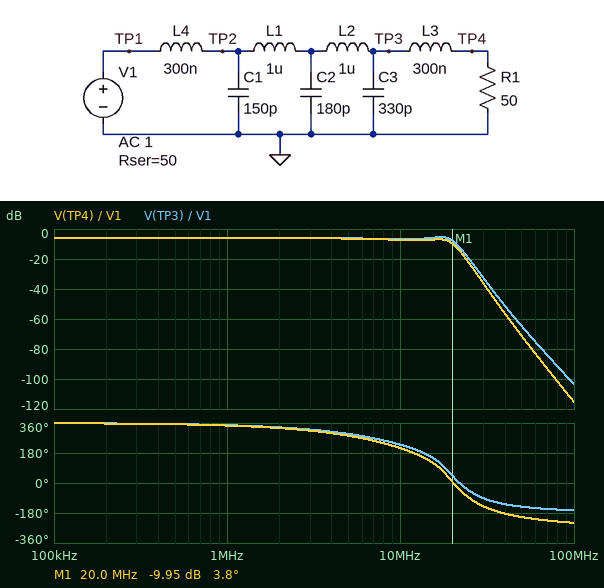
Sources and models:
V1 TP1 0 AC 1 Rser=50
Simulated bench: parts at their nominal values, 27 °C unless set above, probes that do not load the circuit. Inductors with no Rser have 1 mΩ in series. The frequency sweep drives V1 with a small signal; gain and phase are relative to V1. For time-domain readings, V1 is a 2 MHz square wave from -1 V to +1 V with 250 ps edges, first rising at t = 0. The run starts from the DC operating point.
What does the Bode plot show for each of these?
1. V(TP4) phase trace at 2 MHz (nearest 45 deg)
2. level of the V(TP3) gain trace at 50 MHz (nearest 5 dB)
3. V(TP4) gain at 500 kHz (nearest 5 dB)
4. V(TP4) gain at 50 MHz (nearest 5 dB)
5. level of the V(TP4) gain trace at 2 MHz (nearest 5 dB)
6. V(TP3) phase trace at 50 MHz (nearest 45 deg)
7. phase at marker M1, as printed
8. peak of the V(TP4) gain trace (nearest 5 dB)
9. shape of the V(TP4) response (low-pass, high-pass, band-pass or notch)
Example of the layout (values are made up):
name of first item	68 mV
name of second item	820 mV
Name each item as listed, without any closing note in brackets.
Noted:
V(TP4) phase trace at 2 MHz	315 deg
level of the V(TP3) gain trace at 50 MHz	-65 dB
V(TP4) gain at 500 kHz	-5 dB
V(TP4) gain at 50 MHz	-70 dB
level of the V(TP4) gain trace at 2 MHz	-5 dB
V(TP3) phase trace at 50 MHz	-135 deg
phase at marker M1, as printed	3.8 deg
peak of the V(TP4) gain trace	-5 dB
shape of the V(TP4) response	low-pass
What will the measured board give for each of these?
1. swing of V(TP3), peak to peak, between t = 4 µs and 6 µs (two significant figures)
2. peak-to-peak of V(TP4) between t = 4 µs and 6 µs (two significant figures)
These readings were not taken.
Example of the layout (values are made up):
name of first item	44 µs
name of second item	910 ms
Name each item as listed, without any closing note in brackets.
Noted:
swing of V(TP3), peak to peak, between t = 4 µs and 6 µs	1.3 V
peak-to-peak of V(TP4) between t = 4 µs and 6 µs	1.2 V
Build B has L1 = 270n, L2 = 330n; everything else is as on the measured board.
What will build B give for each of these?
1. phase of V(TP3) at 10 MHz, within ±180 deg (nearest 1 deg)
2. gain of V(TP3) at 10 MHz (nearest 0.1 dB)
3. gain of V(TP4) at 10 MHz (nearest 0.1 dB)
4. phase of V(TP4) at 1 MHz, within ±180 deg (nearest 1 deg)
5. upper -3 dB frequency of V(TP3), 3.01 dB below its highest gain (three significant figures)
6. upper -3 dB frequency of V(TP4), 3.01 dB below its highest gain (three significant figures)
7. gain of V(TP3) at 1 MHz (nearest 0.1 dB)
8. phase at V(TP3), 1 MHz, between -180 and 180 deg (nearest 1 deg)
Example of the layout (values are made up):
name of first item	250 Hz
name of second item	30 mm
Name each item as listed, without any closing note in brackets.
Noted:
phase of V(TP3) at 10 MHz, within ±180 deg	-83 deg
gain of V(TP3) at 10 MHz	-6.1 dB
gain of V(TP4) at 10 MHz	-6.7 dB
phase of V(TP4) at 1 MHz, within ±180 deg	-10 deg
upper -3 dB frequency of V(TP3), 3.01 dB below its highest gain	26.8 MHz
upper -3 dB frequency of V(TP4), 3.01 dB below its highest gain	25.7 MHz
gain of V(TP3) at 1 MHz	-6.0 dB
phase at V(TP3), 1 MHz, between -180 and 180 deg	-8 deg
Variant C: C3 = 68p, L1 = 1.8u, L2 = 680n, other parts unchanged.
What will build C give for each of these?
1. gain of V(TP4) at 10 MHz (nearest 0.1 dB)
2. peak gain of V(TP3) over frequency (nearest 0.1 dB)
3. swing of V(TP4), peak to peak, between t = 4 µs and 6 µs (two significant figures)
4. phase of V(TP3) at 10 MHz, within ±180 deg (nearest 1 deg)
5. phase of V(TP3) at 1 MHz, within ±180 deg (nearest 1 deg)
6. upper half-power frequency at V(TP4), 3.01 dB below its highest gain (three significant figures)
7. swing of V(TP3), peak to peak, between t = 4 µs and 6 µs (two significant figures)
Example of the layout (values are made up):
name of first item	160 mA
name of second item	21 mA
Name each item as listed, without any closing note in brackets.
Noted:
gain of V(TP4) at 10 MHz	-7.4 dB
peak gain of V(TP3) over frequency	-6.0 dB
swing of V(TP4), peak to peak, between t = 4 µs and 6 µs	1.0 V
phase of V(TP3) at 10 MHz, within ±180 deg	-106 deg
phase of V(TP3) at 1 MHz, within ±180 deg	-12 deg
upper half-power frequency at V(TP4), 3.01 dB below its highest gain	16.4 MHz
swing of V(TP3), peak to peak, between t = 4 µs and 6 µs	1.1 V
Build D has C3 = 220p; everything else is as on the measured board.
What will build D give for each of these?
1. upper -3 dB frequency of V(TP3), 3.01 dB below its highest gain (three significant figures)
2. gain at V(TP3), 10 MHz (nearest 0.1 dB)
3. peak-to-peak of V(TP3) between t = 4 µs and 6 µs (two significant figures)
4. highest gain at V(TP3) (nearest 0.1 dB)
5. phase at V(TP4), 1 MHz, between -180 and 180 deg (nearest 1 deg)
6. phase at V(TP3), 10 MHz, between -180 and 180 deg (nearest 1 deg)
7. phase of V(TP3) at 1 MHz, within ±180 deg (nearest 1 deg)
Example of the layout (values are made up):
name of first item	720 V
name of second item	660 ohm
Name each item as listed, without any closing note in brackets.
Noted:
upper -3 dB frequency of V(TP3), 3.01 dB below its highest gain	21.7 MHz
gain at V(TP3), 10 MHz	-6.1 dB
peak-to-peak of V(TP3) between t = 4 µs and 6 µs	1.4 V
highest gain at V(TP3)	-4.5 dB
phase at V(TP4), 1 MHz, between -180 and 180 deg	-14 deg
phase at V(TP3), 10 MHz, between -180 and 180 deg	-117 deg
phase of V(TP3) at 1 MHz, within ±180 deg	-12 deg
